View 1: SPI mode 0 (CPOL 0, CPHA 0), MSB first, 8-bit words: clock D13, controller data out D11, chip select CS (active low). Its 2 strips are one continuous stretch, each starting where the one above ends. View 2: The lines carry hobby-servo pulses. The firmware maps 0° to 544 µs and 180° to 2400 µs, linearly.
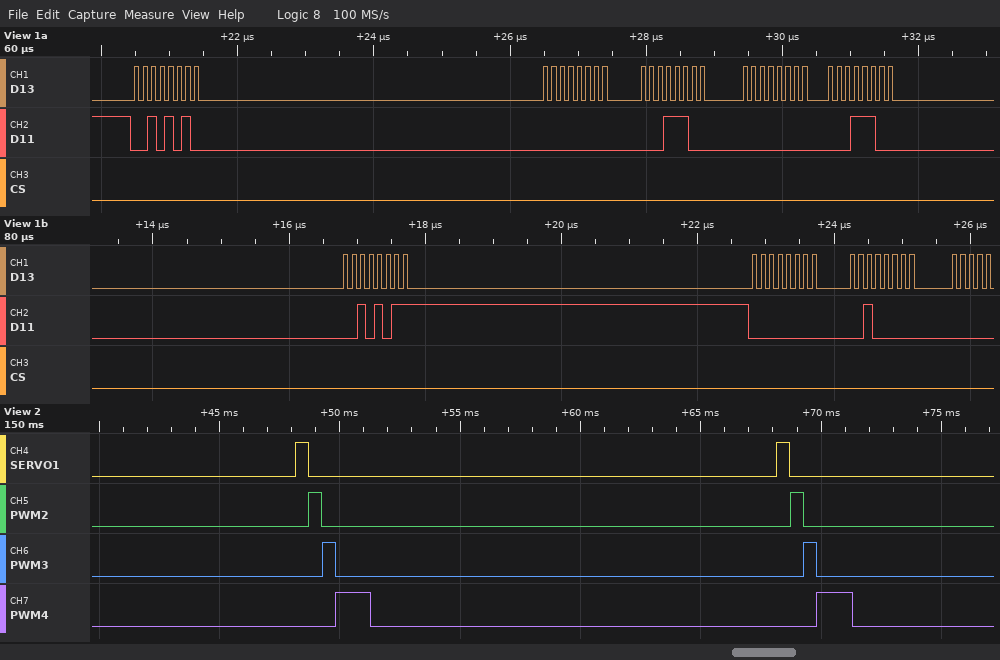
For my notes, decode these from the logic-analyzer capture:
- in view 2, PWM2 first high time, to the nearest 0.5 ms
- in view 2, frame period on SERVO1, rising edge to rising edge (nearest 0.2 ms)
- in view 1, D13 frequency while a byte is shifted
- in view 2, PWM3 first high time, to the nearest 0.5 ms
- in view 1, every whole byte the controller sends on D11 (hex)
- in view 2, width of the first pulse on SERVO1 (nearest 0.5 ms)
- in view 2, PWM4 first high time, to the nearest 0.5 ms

0.5 ms
20.0 ms
8 MHz
0.5 ms
0x2A 0x00 0x1C 0x00 0x1C 0x2B 0x00 0x20
0.5 ms
1.5 ms
